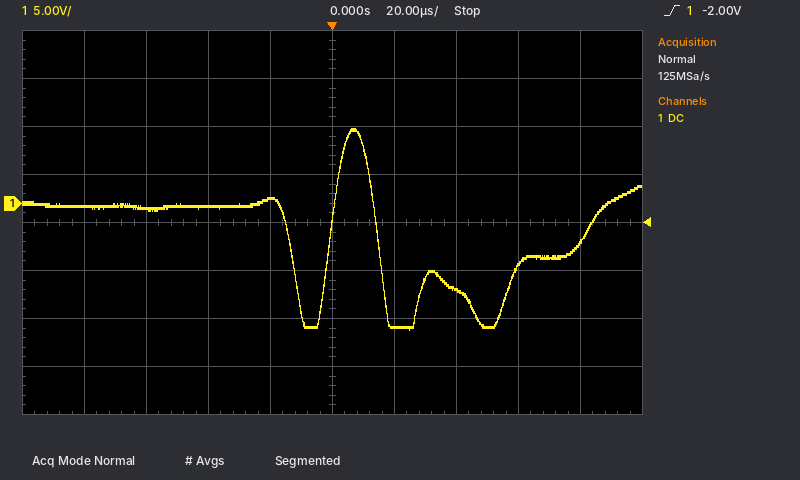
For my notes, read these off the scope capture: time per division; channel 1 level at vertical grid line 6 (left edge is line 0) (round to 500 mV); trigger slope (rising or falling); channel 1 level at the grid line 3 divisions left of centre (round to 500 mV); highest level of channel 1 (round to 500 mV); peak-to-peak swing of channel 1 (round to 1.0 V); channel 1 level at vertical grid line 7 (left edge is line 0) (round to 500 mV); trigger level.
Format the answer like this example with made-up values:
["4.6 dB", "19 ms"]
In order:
["20 µs", "-13.0 V", "rising", "-500 mV", "8.0 V", "21.0 V", "-9.0 V", "-2.00 V"]
